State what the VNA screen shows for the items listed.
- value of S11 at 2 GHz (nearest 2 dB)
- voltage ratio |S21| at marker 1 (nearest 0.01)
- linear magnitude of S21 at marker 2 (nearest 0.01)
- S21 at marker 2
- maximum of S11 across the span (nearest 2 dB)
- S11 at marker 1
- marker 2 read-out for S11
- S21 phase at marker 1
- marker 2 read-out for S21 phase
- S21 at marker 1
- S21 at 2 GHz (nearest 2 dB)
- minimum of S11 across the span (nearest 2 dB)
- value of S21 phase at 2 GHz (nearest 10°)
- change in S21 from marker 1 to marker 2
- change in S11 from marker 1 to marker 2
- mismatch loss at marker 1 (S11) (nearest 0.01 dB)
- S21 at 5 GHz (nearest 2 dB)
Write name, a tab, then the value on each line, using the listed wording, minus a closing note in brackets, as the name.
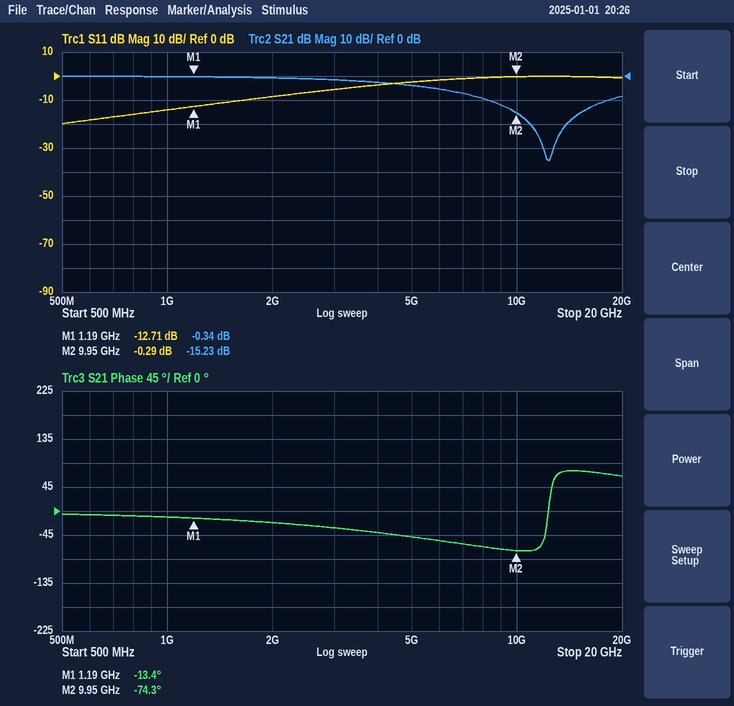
value of S11 at 2 GHz	-8 dB
voltage ratio |S21| at marker 1	0.96
linear magnitude of S21 at marker 2	0.17
S21 at marker 2	-15.23 dB
maximum of S11 across the span	0 dB
S11 at marker 1	-12.71 dB
marker 2 read-out for S11	-0.29 dB
S21 phase at marker 1	-13.4°
marker 2 read-out for S21 phase	-74.3°
S21 at marker 1	-0.34 dB
S21 at 2 GHz	0 dB
minimum of S11 across the span	-20 dB
value of S21 phase at 2 GHz	-20°
change in S21 from marker 1 to marker 2	-14.89 dB
change in S11 from marker 1 to marker 2	12.42 dB
mismatch loss at marker 1 (S11)	0.24 dB
S21 at 5 GHz	-4 dB
